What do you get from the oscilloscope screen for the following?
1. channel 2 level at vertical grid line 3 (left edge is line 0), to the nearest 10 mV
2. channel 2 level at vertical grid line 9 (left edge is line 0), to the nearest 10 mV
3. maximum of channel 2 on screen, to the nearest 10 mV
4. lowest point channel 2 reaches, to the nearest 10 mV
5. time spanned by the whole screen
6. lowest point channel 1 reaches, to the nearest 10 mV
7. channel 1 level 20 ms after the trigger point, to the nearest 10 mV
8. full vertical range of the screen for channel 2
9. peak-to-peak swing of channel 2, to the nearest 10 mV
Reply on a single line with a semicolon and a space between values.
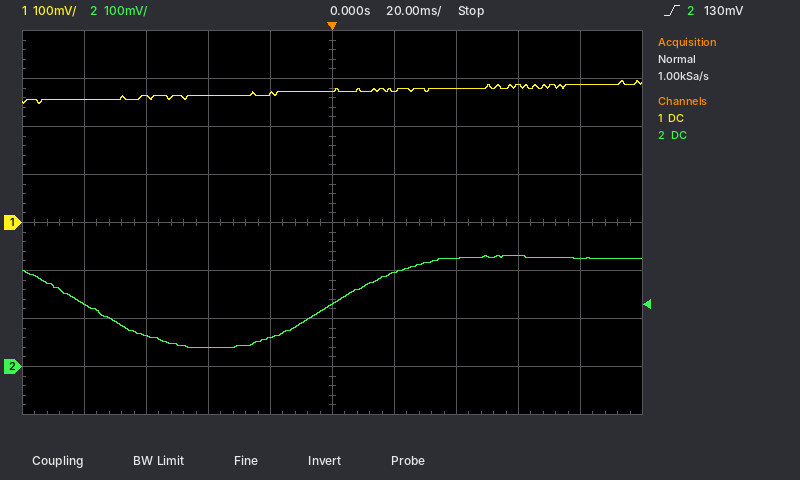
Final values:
40 mV; 220 mV; 230 mV; 40 mV; 200 ms; 250 mV; 270 mV; 800 mV; 190 mV
